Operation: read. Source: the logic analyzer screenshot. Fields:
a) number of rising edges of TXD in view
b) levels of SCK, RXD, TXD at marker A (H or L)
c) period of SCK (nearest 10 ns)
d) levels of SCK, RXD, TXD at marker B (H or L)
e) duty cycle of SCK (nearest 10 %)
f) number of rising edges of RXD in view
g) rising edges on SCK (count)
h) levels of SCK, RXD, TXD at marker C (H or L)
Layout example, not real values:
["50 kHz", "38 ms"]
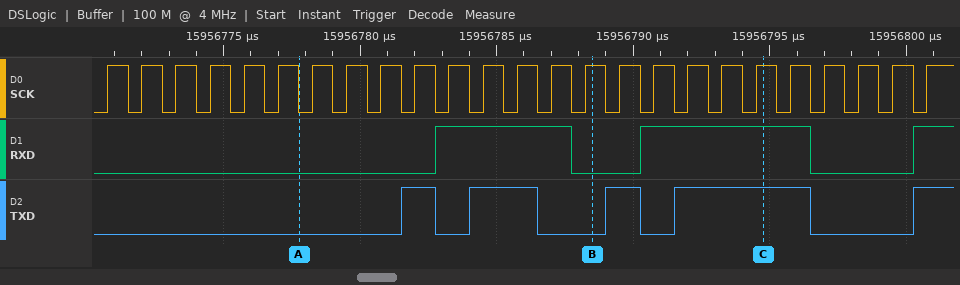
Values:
["5", "SCK=L, RXD=L, TXD=L", "1250 ns", "SCK=H, RXD=L, TXD=L", "60 %", "3", "25", "SCK=H, RXD=H, TXD=H"]
